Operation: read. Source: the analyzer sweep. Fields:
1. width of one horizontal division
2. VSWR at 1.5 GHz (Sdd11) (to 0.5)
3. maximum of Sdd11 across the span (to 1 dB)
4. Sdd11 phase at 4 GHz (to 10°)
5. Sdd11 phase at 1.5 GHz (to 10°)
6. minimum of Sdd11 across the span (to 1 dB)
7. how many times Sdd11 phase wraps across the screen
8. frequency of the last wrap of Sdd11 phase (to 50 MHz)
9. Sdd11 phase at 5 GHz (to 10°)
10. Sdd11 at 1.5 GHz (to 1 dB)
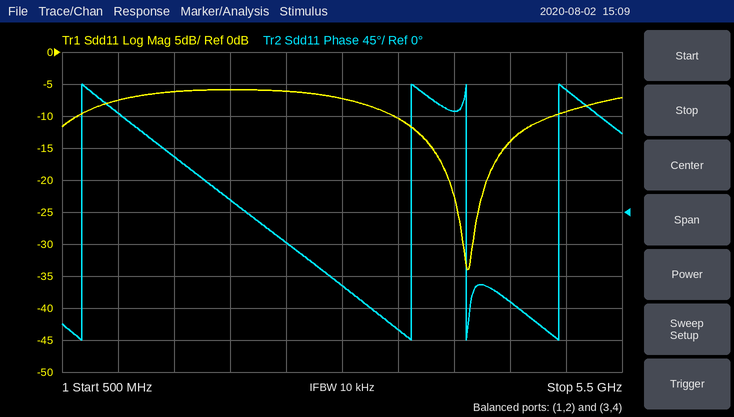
500 MHz
3.0
-6 dB
140°
80°
-34 dB
4
4.95 GHz
170°
-6 dB
